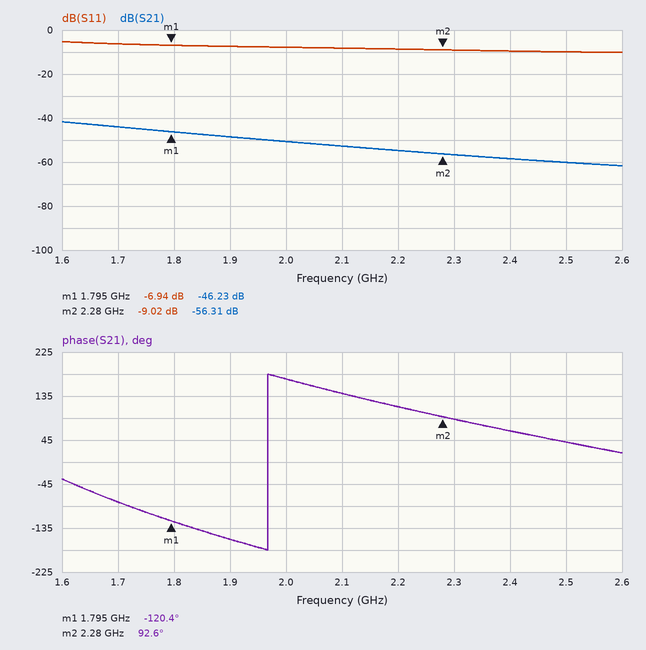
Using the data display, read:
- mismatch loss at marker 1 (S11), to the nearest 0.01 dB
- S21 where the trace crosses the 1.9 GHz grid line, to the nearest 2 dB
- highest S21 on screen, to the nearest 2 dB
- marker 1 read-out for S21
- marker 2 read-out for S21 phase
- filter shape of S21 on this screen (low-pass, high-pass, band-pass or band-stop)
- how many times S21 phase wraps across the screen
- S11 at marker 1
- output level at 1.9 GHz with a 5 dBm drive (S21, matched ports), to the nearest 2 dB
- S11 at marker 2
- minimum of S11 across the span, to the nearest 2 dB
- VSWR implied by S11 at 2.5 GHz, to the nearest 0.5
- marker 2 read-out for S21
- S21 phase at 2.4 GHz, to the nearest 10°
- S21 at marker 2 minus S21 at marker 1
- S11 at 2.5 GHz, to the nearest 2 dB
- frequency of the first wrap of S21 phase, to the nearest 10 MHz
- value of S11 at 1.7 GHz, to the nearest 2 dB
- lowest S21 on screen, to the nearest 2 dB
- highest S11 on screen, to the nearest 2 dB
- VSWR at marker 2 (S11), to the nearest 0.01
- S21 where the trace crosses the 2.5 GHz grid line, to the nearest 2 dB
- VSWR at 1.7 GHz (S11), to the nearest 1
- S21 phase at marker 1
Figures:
0.98 dB
-48 dB
-42 dB
-46.23 dB
92.6°
low-pass
1
-6.94 dB
-44 dBm
-9.02 dB
-10 dB
2.0
-56.31 dB
60°
-10.08 dB
-10 dB
1.97 GHz
-6 dB
-62 dB
-6 dB
2.10
-60 dB
3
-120.4°
